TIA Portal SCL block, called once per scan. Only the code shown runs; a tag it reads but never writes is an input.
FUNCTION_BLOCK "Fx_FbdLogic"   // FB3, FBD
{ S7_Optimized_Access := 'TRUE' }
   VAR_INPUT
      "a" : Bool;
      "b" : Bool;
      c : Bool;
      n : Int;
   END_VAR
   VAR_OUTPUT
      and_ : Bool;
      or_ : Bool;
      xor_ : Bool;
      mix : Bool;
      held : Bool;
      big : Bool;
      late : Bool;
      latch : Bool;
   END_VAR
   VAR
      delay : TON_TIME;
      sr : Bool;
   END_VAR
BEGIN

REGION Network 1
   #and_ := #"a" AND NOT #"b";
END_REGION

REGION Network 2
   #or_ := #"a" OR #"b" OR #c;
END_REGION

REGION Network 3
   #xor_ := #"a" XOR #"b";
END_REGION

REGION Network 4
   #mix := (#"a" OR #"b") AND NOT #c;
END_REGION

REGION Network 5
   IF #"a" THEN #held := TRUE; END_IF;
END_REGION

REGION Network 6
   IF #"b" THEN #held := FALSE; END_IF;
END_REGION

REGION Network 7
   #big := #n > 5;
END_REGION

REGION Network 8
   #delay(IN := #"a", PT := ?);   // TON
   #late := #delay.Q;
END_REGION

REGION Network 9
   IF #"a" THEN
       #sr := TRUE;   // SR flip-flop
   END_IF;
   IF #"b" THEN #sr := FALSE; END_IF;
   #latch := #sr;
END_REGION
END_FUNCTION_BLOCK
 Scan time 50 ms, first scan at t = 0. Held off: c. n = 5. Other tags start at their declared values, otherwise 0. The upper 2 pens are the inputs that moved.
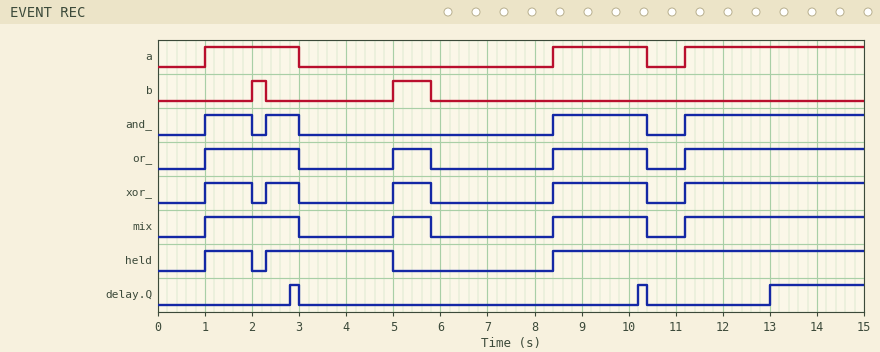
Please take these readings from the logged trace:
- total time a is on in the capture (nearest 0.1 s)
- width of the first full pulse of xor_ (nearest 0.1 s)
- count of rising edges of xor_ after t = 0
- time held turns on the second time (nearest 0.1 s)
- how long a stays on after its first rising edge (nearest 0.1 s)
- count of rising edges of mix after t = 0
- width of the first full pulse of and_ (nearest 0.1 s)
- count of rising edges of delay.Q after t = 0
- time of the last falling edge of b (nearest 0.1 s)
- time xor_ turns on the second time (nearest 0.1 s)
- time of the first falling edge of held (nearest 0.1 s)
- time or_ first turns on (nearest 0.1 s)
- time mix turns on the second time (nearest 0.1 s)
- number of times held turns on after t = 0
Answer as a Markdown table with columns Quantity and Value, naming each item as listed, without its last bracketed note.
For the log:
| Quantity | Value |
|---|---|
| total time a is on in the capture | 7.8 s |
| width of the first full pulse of xor_ | 1.0 s |
| count of rising edges of xor_ after t = 0 | 5 |
| time held turns on the second time | 2.3 s |
| how long a stays on after its first rising edge | 2.0 s |
| count of rising edges of mix after t = 0 | 4 |
| width of the first full pulse of and_ | 1.0 s |
| count of rising edges of delay.Q after t = 0 | 3 |
| time of the last falling edge of b | 5.8 s |
| time xor_ turns on the second time | 2.3 s |
| time of the first falling edge of held | 2.0 s |
| time or_ first turns on | 1.0 s |
| time mix turns on the second time | 5.0 s |
| number of times held turns on after t = 0 | 3 |
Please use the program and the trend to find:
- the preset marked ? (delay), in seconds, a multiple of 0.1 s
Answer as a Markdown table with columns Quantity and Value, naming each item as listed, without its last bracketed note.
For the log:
| Quantity | Value |
|---|---|
| the preset marked ? (delay), in seconds, a multiple of 0.1 s | 1.8 s |
